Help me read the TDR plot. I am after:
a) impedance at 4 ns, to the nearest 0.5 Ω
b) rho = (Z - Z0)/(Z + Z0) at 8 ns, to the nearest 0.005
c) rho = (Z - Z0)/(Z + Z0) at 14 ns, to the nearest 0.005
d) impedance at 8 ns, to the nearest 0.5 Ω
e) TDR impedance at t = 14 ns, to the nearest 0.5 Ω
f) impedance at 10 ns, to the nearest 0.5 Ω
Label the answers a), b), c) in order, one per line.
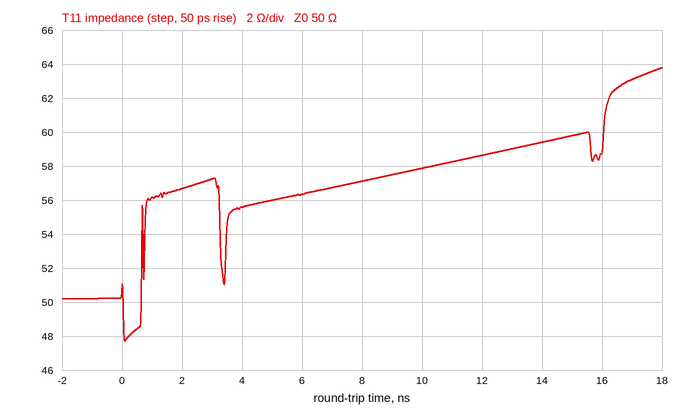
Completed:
a) 55.5 Ω
b) +0.065
c) +0.085
d) 57.0 Ω
e) 59.5 Ω
f) 58.0 Ω
